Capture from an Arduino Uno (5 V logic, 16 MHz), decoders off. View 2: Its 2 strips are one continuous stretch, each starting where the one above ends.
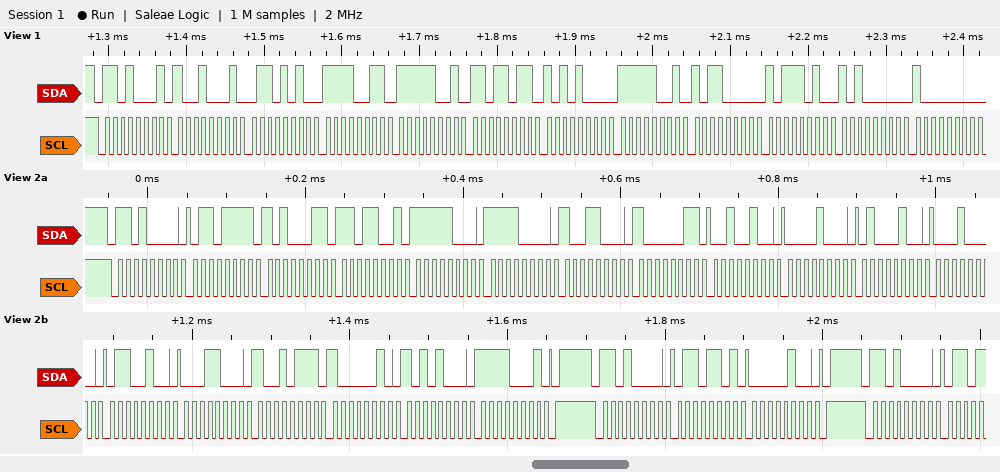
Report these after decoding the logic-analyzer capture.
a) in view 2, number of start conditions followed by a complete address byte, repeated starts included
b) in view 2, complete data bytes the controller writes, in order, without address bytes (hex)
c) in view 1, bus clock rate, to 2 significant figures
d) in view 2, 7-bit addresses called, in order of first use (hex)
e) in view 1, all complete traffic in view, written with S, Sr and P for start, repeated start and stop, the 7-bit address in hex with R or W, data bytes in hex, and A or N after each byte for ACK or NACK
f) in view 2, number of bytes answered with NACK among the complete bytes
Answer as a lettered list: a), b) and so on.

a) 3
b) 6F A3 D9 F8 F0 98 83 24 08 44 10 64 18 97 82 A8 F1 6D 04
c) 100 kHz
d) 0x68
e) S 68R A 91 A 6A A F3 A F9 A DB A A8 A F9 A B0 A BA A A0 A 80 A
f) 0
